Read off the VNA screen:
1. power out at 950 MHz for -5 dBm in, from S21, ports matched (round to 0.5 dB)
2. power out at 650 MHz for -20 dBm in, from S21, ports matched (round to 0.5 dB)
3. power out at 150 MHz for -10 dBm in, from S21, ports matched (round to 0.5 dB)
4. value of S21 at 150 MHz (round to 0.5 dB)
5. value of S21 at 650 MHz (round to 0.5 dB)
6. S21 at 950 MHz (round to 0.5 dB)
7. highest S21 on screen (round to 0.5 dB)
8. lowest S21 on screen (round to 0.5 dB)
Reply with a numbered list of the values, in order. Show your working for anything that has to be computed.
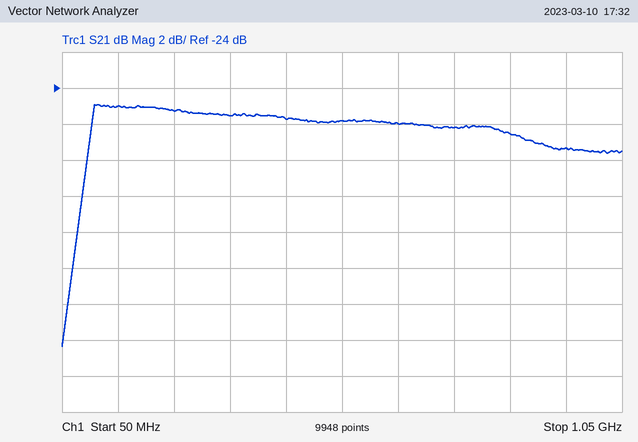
1. -5 dBm + (-27.5 dB) = -32.5 dBm
2. -20 dBm + (-26.0 dB) = -46.0 dBm
3. -10 dBm + (-25.0 dB) = -35.0 dBm
4. -25.0 dB
5. -26.0 dB
6. -27.5 dB
7. -25.0 dB
8. -38.5 dB
